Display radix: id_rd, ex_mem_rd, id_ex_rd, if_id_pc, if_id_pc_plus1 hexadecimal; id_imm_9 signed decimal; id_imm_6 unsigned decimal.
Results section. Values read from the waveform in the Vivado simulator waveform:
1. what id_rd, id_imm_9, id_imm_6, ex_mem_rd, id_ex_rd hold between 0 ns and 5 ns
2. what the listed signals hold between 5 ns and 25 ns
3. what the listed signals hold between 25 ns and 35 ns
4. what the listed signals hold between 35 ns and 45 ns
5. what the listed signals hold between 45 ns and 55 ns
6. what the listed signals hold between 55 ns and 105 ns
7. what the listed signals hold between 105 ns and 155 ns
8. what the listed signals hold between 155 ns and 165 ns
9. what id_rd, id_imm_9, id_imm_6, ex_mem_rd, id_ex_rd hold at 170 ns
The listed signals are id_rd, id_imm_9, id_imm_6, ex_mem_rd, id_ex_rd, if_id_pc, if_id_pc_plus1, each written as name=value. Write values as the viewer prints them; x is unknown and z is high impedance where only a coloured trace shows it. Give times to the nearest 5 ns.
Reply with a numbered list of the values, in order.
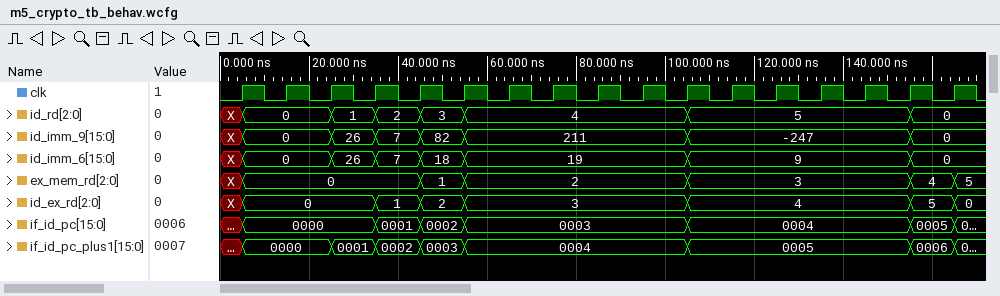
1. id_rd=X, id_imm_9=X, id_imm_6=X, ex_mem_rd=X, id_ex_rd=X
2. id_rd=0, id_imm_9=0, id_imm_6=0, ex_mem_rd=0, id_ex_rd=0, if_id_pc=0000, if_id_pc_plus1=0000
3. id_rd=1, id_imm_9=26, id_imm_6=26, ex_mem_rd=0, id_ex_rd=0, if_id_pc=0000, if_id_pc_plus1=0001
4. id_rd=2, id_imm_9=7, id_imm_6=7, ex_mem_rd=0, id_ex_rd=1, if_id_pc=0001, if_id_pc_plus1=0002
5. id_rd=3, id_imm_9=82, id_imm_6=18, ex_mem_rd=1, id_ex_rd=2, if_id_pc=0002, if_id_pc_plus1=0003
6. id_rd=4, id_imm_9=211, id_imm_6=19, ex_mem_rd=2, id_ex_rd=3, if_id_pc=0003, if_id_pc_plus1=0004
7. id_rd=5, id_imm_9=-247, id_imm_6=9, ex_mem_rd=3, id_ex_rd=4, if_id_pc=0004, if_id_pc_plus1=0005
8. id_rd=0, id_imm_9=0, id_imm_6=0, ex_mem_rd=4, id_ex_rd=5, if_id_pc=0005, if_id_pc_plus1=0006
9. id_rd=0, id_imm_9=0, id_imm_6=0, ex_mem_rd=5, id_ex_rd=0
